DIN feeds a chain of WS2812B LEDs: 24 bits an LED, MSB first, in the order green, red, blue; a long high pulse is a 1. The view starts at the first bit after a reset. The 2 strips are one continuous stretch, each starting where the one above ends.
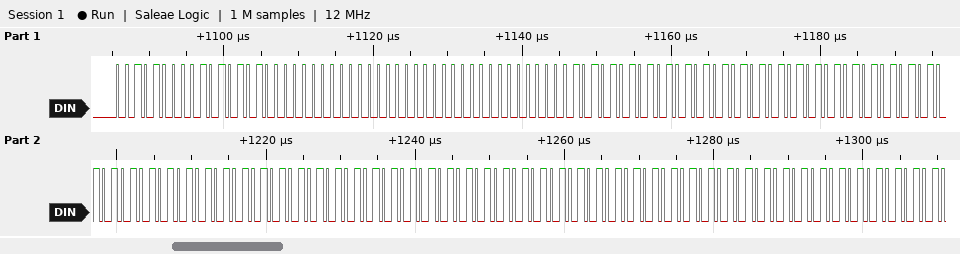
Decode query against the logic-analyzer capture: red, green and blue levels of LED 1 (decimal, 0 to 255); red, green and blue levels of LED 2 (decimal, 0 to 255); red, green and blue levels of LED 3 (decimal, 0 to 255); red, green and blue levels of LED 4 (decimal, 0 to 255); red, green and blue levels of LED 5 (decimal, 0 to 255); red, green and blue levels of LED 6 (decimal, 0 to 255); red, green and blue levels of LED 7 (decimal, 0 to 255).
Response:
85, 40, 0
0, 0, 0
85, 85, 85
85, 85, 85
85, 85, 85
85, 85, 85
85, 85, 85
